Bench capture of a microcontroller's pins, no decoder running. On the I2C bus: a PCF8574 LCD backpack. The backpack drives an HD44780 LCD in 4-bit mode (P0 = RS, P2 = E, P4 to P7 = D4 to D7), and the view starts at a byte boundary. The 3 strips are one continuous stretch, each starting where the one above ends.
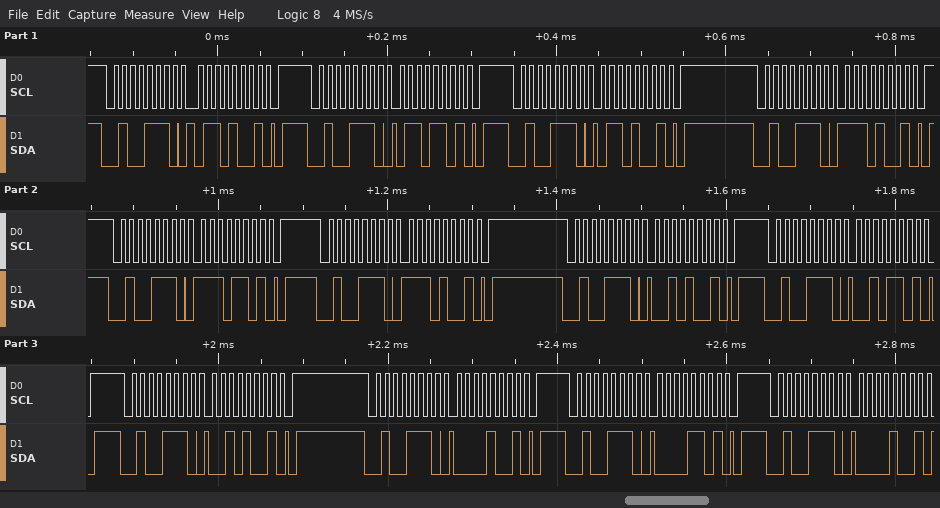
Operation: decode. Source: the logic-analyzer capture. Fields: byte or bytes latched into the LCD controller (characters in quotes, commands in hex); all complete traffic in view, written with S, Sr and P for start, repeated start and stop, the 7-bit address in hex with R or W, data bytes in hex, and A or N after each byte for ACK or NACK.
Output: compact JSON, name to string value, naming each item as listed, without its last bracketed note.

{"byte or bytes latched into the LCD controller": "'n' ' '", "all complete traffic in view, written with S, Sr and P for start, repeated start and stop, the 7-bit address in hex with R or W, data bytes in hex, and A or N after each byte for ACK or NACK": "S 27W A 69 A P S 27W A 6D A P S 27W A 69 A P S 27W A E9 A P S 27W A ED A P S 27W A E9 A P S 27W A 29 A P S 27W A 2D A P S 27W A 29 A P S 27W A 09 A P S 27W A 0D A P S 27W A 09 A"}
